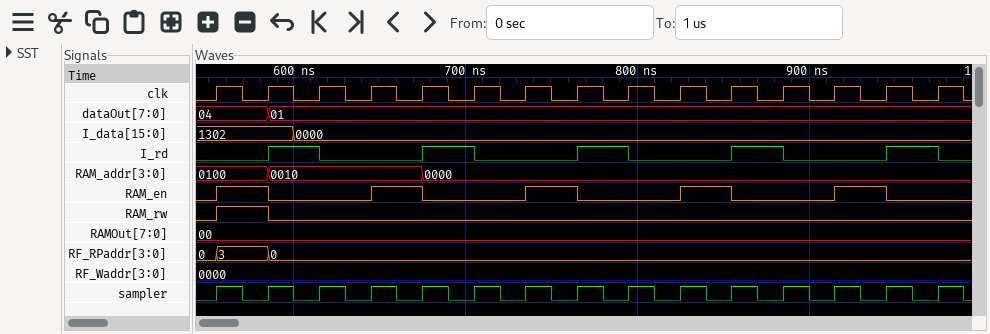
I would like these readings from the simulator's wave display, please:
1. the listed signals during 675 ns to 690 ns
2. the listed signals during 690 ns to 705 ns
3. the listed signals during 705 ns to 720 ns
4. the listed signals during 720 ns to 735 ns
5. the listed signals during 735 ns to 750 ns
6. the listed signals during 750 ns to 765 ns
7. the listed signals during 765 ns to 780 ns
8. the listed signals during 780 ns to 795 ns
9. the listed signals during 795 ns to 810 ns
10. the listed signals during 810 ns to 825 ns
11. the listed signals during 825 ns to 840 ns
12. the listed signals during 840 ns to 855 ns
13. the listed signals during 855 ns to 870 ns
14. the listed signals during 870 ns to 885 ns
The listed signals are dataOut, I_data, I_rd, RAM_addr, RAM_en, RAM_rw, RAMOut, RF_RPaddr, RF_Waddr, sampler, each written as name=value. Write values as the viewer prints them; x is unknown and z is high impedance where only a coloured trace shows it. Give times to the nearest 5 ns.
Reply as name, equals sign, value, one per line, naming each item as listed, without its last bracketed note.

the listed signals during 675 ns to 690 ns = dataOut=01, I_data=0000, I_rd=1, RAM_addr=0000, RAM_en=0, RAM_rw=0, RAMOut=00, RF_RPaddr=0, RF_Waddr=0000, sampler=1
the listed signals during 690 ns to 705 ns = dataOut=01, I_data=0000, I_rd=1, RAM_addr=0000, RAM_en=0, RAM_rw=0, RAMOut=00, RF_RPaddr=0, RF_Waddr=0000, sampler=0
the listed signals during 705 ns to 720 ns = dataOut=01, I_data=0000, I_rd=0, RAM_addr=0000, RAM_en=0, RAM_rw=0, RAMOut=00, RF_RPaddr=0, RF_Waddr=0000, sampler=1
the listed signals during 720 ns to 735 ns = dataOut=01, I_data=0000, I_rd=0, RAM_addr=0000, RAM_en=0, RAM_rw=0, RAMOut=00, RF_RPaddr=0, RF_Waddr=0000, sampler=0
the listed signals during 735 ns to 750 ns = dataOut=01, I_data=0000, I_rd=0, RAM_addr=0000, RAM_en=1, RAM_rw=0, RAMOut=00, RF_RPaddr=0, RF_Waddr=0000, sampler=1
the listed signals during 750 ns to 765 ns = dataOut=01, I_data=0000, I_rd=0, RAM_addr=0000, RAM_en=1, RAM_rw=0, RAMOut=00, RF_RPaddr=0, RF_Waddr=0000, sampler=0
the listed signals during 765 ns to 780 ns = dataOut=01, I_data=0000, I_rd=1, RAM_addr=0000, RAM_en=0, RAM_rw=0, RAMOut=00, RF_RPaddr=0, RF_Waddr=0000, sampler=1
the listed signals during 780 ns to 795 ns = dataOut=01, I_data=0000, I_rd=1, RAM_addr=0000, RAM_en=0, RAM_rw=0, RAMOut=00, RF_RPaddr=0, RF_Waddr=0000, sampler=0
the listed signals during 795 ns to 810 ns = dataOut=01, I_data=0000, I_rd=0, RAM_addr=0000, RAM_en=0, RAM_rw=0, RAMOut=00, RF_RPaddr=0, RF_Waddr=0000, sampler=1
the listed signals during 810 ns to 825 ns = dataOut=01, I_data=0000, I_rd=0, RAM_addr=0000, RAM_en=0, RAM_rw=0, RAMOut=00, RF_RPaddr=0, RF_Waddr=0000, sampler=0
the listed signals during 825 ns to 840 ns = dataOut=01, I_data=0000, I_rd=0, RAM_addr=0000, RAM_en=1, RAM_rw=0, RAMOut=00, RF_RPaddr=0, RF_Waddr=0000, sampler=1
the listed signals during 840 ns to 855 ns = dataOut=01, I_data=0000, I_rd=0, RAM_addr=0000, RAM_en=1, RAM_rw=0, RAMOut=00, RF_RPaddr=0, RF_Waddr=0000, sampler=0
the listed signals during 855 ns to 870 ns = dataOut=01, I_data=0000, I_rd=1, RAM_addr=0000, RAM_en=0, RAM_rw=0, RAMOut=00, RF_RPaddr=0, RF_Waddr=0000, sampler=1
the listed signals during 870 ns to 885 ns = dataOut=01, I_data=0000, I_rd=1, RAM_addr=0000, RAM_en=0, RAM_rw=0, RAMOut=00, RF_RPaddr=0, RF_Waddr=0000, sampler=0
